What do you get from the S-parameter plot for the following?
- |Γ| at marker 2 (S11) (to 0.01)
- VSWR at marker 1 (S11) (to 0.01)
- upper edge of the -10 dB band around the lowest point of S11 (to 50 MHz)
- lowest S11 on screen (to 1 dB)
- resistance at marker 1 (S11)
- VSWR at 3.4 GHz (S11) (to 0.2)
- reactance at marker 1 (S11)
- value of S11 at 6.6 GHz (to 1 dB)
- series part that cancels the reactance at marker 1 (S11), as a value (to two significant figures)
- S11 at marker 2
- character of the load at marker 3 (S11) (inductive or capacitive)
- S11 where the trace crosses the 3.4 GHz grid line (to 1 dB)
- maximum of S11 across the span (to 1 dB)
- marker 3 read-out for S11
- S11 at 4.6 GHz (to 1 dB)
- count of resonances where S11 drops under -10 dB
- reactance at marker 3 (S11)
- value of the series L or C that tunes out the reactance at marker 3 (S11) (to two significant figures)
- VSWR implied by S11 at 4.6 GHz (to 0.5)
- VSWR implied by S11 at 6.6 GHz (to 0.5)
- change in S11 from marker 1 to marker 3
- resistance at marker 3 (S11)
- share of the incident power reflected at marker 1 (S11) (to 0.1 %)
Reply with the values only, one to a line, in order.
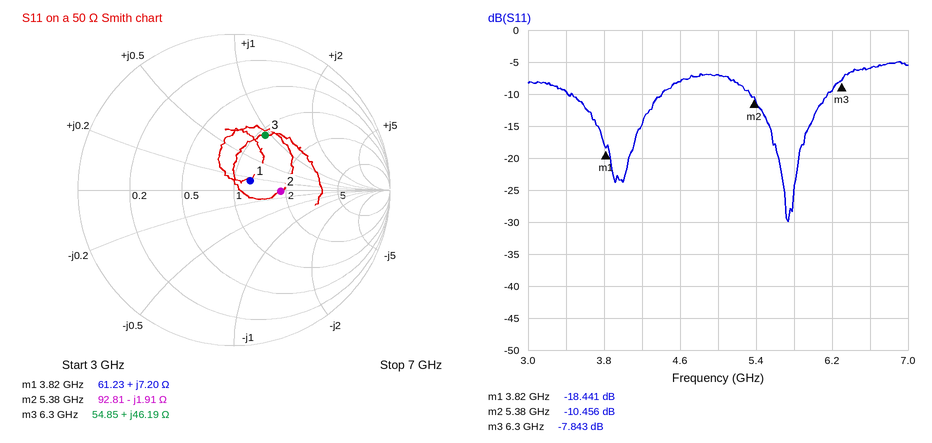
0.30
1.27
6.15 GHz
-30 dB
61.23 Ω
2.0
+7.20 Ω
-6 dB
5.8 pF
-10.456 dB
inductive
-10 dB
-5 dB
-7.843 dB
-8 dB
2
+46.19 Ω
550 fF
2.5
3.0
10.598 dB
54.85 Ω
1.4 %
